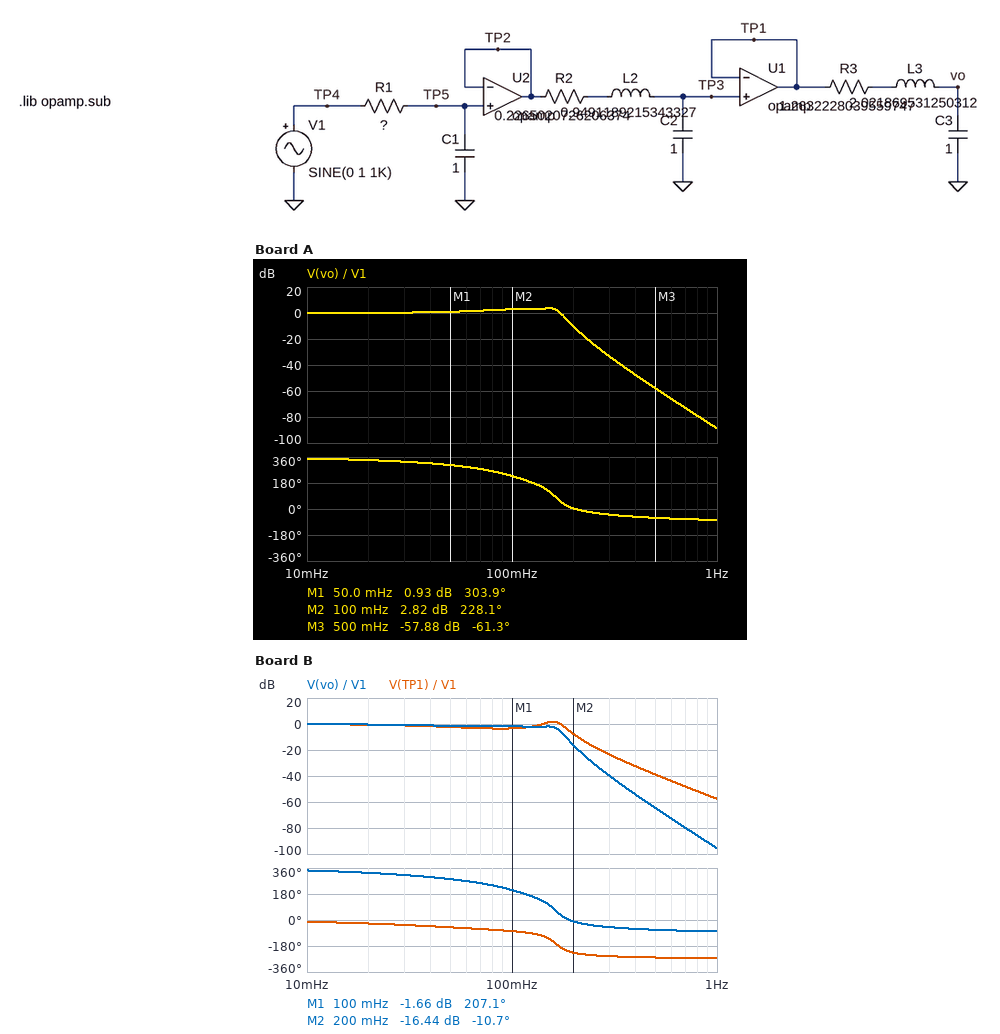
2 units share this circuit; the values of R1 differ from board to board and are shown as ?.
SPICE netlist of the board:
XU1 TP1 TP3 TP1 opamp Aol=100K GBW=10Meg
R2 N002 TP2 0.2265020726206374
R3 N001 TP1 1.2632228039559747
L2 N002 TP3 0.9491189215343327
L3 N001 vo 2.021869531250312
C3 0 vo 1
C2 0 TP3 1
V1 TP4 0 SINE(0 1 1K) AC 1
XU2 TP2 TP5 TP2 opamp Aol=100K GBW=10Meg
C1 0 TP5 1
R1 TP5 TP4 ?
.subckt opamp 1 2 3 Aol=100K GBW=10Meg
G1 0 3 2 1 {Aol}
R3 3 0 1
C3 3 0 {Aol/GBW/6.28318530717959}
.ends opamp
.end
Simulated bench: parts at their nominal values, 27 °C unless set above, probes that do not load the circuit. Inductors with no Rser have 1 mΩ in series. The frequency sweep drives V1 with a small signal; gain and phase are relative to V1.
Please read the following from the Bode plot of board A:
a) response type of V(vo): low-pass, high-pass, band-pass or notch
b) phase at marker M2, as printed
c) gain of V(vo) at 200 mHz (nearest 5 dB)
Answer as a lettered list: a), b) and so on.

a) low-pass
b) 228.1 deg
c) -10 dB
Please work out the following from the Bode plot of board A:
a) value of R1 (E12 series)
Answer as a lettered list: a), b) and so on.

a) 1.5 Ω
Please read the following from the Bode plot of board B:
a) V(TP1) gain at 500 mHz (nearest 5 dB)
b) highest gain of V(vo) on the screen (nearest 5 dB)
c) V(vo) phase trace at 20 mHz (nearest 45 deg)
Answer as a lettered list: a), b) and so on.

a) -40 dB
b) 0 dB
c) 315 deg
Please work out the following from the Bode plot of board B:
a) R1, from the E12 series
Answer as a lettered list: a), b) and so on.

a) 3.3 Ω
